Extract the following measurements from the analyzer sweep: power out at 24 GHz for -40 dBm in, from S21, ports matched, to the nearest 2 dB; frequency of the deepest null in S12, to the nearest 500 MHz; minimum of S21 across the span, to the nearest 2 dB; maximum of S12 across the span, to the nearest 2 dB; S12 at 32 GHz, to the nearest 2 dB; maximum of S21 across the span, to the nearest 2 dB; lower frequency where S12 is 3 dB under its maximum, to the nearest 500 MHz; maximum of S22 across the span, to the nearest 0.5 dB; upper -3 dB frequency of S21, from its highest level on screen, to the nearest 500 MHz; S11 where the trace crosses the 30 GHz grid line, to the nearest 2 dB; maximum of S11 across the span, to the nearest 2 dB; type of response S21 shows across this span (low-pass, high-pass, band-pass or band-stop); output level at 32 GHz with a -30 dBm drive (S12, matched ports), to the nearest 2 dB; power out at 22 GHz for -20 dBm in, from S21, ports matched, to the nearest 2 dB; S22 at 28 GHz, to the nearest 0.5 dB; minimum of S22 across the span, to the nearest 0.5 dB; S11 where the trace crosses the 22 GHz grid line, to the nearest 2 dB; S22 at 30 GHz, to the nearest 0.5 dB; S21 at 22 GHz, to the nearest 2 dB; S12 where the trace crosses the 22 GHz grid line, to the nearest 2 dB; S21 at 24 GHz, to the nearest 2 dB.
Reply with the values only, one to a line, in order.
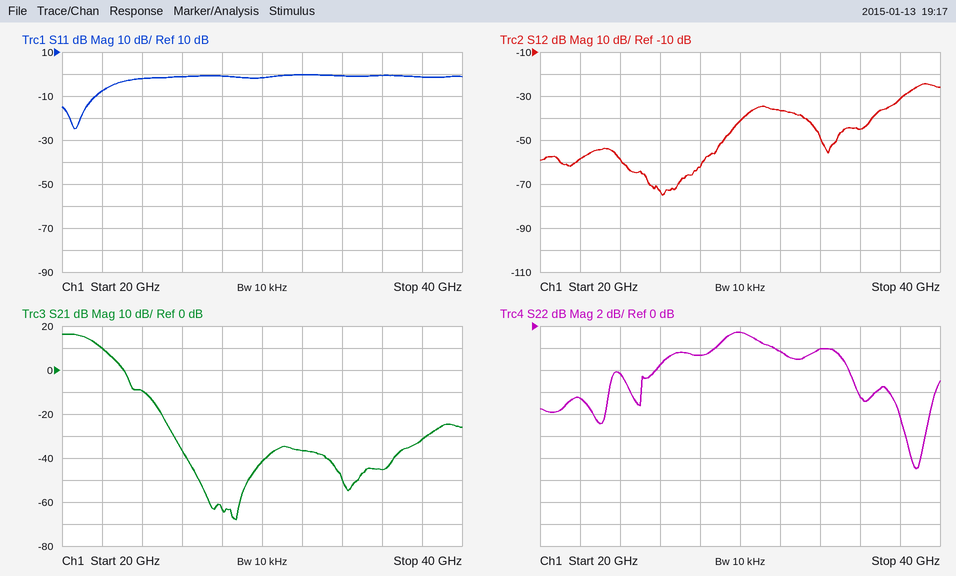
-50 dBm
26.0 GHz
-68 dB
-24 dB
-36 dB
16 dB
38.5 GHz
-0.5 dB
21.5 GHz
-2 dB
0 dB
low-pass
-66 dBm
-10 dBm
-2.5 dB
-13.0 dB
-8 dB
-0.5 dB
10 dB
-58 dB
-10 dB
